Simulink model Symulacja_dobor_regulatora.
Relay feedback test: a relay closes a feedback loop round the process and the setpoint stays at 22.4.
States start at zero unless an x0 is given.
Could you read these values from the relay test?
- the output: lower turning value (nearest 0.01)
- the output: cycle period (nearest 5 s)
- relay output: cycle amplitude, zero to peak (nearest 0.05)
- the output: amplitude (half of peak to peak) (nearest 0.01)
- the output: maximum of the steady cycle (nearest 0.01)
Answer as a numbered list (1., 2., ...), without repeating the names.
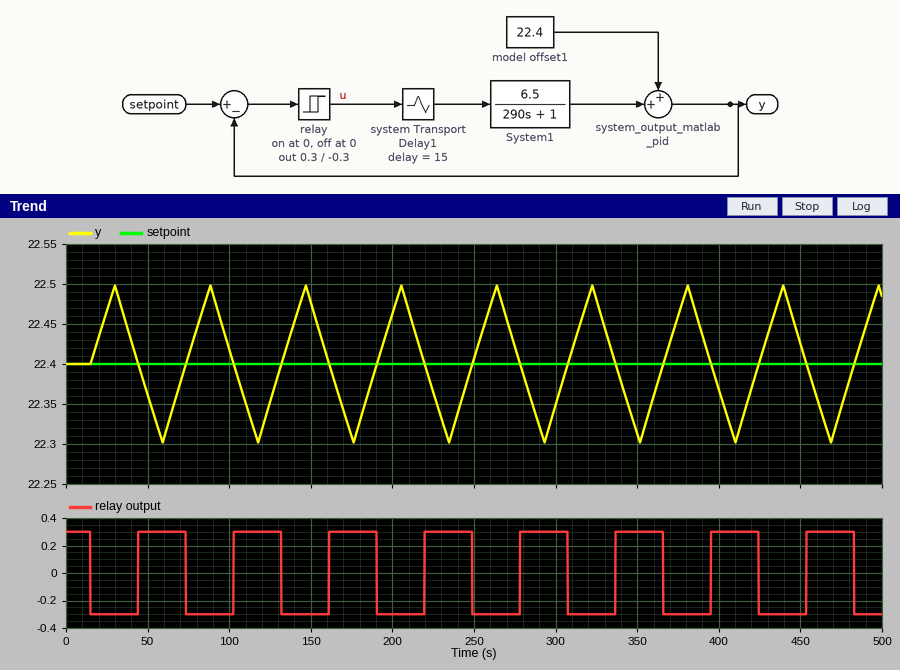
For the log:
1. 22.30
2. 60 s
3. 0.30
4. 0.10
5. 22.50
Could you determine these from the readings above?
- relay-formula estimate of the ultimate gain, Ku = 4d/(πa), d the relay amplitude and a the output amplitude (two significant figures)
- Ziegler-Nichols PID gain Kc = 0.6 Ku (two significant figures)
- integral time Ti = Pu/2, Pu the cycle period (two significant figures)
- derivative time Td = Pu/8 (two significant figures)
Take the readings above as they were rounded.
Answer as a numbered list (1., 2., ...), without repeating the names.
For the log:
1. 3.8
2. 2.3
3. 30 s
4. 7.5 s
